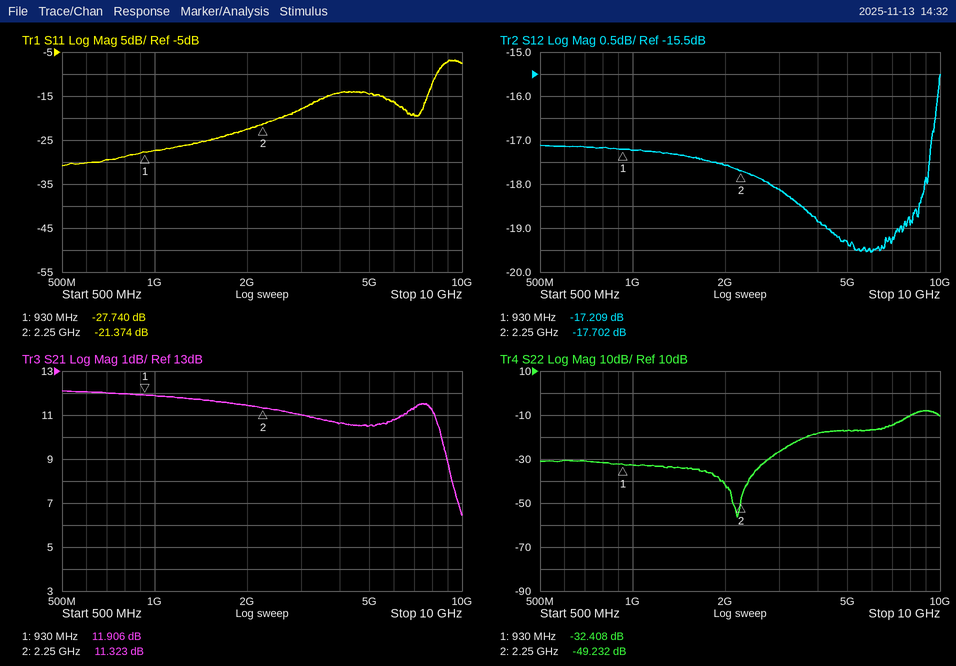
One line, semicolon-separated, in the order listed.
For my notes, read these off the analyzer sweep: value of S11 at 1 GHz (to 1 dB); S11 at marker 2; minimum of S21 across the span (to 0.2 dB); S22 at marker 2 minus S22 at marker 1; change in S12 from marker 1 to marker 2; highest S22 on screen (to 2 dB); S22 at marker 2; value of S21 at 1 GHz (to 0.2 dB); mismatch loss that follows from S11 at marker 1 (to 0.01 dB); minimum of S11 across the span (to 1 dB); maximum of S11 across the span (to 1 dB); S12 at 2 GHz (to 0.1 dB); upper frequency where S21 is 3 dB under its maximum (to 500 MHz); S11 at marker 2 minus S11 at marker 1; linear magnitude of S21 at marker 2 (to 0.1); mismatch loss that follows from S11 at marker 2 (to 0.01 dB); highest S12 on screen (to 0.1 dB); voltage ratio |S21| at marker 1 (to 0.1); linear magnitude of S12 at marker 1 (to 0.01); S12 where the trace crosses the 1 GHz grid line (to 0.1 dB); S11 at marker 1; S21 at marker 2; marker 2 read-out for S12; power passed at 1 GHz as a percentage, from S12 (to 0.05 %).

-27 dB; -21.374 dB; 6.4 dB; -16.824 dB; -0.493 dB; -8 dB; -49.232 dB; 11.8 dB; 0.01 dB; -31 dB; -7 dB; -17.6 dB; 9.0 GHz; 6.366 dB; 3.7; 0.03 dB; -15.5 dB; 3.9; 0.14; -17.2 dB; -27.740 dB; 11.323 dB; -17.702 dB; 1.90 %
